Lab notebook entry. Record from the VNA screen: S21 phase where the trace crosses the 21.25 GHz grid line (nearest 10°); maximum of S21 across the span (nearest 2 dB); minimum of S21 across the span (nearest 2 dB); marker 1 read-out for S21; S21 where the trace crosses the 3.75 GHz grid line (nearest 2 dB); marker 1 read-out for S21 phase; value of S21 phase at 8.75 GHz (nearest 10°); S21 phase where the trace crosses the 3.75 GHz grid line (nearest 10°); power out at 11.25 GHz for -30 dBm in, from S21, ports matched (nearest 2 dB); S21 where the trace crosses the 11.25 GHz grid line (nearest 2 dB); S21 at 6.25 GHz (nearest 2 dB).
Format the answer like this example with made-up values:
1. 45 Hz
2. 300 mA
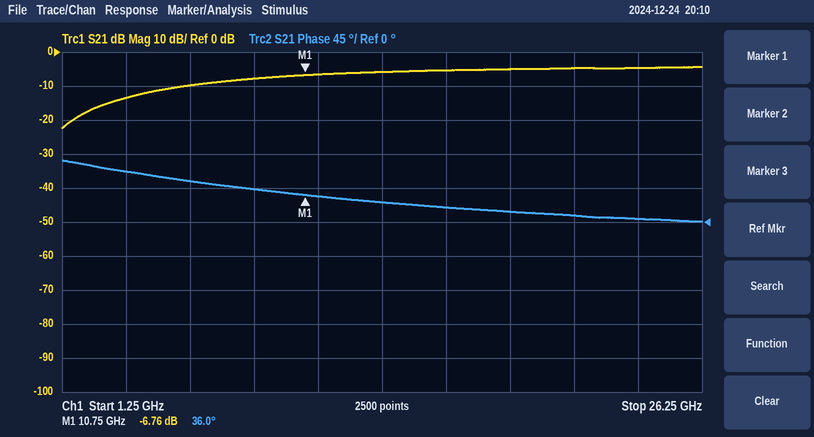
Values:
1. 10°
2. -4 dB
3. -22 dB
4. -6.76 dB
5. -14 dB
6. 36.0°
7. 40°
8. 70°
9. -36 dBm
10. -6 dB
11. -10 dB
